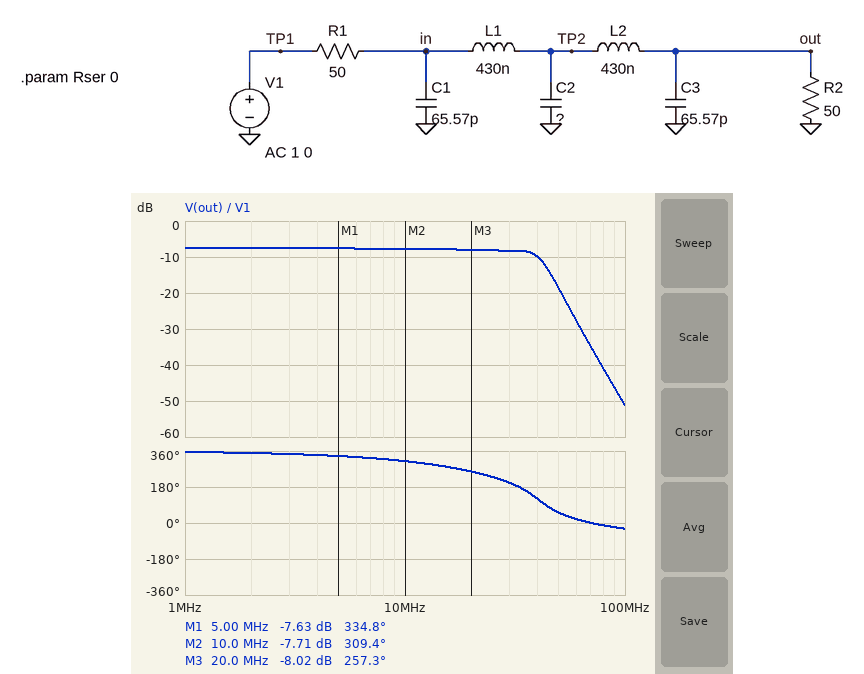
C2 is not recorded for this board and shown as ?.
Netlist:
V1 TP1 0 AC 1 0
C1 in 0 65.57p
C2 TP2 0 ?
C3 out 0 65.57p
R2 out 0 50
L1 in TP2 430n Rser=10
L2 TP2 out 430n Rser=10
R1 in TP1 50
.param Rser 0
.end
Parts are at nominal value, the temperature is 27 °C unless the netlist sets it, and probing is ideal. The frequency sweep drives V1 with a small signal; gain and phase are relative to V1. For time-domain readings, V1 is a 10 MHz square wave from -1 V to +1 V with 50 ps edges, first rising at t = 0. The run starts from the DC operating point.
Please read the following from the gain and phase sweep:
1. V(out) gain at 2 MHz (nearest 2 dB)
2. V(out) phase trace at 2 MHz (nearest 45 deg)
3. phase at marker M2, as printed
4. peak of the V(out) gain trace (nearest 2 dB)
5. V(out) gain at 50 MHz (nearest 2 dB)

-8 dB
360 deg
309.4 deg
-8 dB
-18 dB
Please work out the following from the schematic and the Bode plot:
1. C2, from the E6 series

100 pF
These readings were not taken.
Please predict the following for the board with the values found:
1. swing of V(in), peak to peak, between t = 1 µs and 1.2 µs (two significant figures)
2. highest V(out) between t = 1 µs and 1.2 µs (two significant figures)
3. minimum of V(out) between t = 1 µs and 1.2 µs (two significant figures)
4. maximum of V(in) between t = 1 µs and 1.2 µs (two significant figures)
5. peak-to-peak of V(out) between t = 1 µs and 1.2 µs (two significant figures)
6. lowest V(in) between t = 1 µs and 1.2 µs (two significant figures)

1.6 V
510 mV
-510 mV
800 mV
1.0 V
-800 mV
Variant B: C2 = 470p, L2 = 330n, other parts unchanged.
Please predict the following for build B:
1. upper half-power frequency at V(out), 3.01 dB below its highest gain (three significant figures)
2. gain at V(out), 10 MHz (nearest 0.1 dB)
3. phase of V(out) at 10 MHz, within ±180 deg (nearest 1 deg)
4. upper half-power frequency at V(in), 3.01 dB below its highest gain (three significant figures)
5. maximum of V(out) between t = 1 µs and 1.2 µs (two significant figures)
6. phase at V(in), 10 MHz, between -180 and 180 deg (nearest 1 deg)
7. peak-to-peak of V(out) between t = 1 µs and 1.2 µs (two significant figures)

14.1 MHz
-9.3 dB
-84 deg
69.3 MHz
400 mV
-4 deg
800 mV
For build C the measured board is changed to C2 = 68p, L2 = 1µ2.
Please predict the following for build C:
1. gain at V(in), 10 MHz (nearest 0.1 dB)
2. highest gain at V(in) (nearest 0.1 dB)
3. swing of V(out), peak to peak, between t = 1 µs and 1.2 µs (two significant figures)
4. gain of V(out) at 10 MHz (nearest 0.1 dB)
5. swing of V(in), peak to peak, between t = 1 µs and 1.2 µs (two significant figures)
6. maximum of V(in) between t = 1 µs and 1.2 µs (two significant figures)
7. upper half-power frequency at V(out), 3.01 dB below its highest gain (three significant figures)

-2.2 dB
-1.2 dB
850 mV
-8.8 dB
2.0 V
1.0 V
17.5 MHz
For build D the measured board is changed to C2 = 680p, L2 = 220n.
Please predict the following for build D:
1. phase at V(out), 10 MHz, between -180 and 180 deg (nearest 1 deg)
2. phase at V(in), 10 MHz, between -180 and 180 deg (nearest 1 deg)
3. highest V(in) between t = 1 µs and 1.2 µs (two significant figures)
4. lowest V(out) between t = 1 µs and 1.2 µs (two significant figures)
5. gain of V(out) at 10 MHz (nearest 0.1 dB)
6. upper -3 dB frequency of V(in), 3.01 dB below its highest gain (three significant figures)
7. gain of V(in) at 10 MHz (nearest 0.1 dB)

-92 deg
11 deg
870 mV
-350 mV
-11.2 dB
68.8 MHz
-10.8 dB
